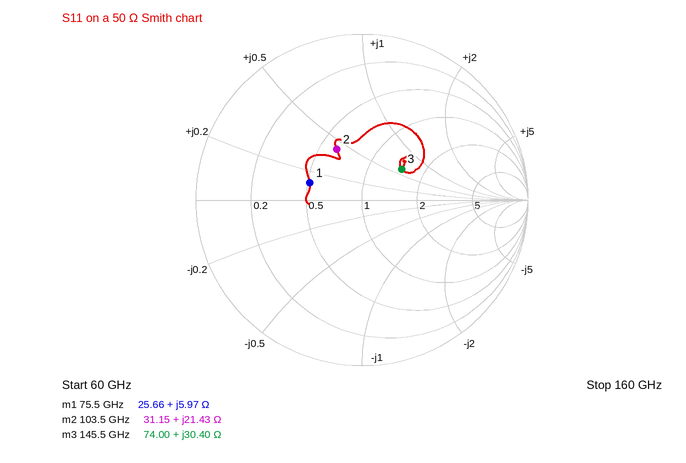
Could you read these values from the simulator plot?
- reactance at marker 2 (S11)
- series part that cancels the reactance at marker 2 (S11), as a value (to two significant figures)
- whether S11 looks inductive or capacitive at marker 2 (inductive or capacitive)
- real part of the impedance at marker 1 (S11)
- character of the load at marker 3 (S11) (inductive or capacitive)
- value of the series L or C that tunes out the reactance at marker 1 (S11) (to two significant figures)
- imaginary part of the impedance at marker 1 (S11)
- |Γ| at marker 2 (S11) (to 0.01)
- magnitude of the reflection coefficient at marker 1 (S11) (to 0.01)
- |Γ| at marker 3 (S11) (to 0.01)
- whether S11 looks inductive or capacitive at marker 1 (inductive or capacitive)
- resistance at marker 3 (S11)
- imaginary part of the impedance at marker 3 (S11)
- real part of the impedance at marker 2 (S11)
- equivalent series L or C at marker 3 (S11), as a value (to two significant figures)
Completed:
+21.43 Ω
72 fF
inductive
25.66 Ω
inductive
350 fF
+5.97 Ω
0.34
0.33
0.30
inductive
74.00 Ω
+30.40 Ω
31.15 Ω
33 pH
